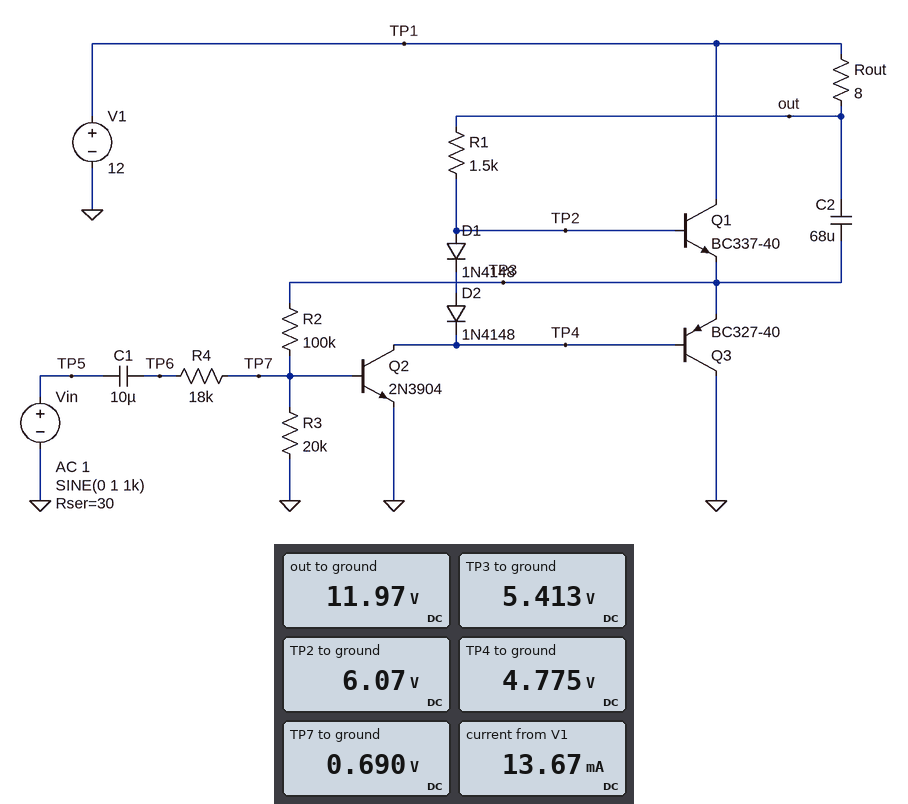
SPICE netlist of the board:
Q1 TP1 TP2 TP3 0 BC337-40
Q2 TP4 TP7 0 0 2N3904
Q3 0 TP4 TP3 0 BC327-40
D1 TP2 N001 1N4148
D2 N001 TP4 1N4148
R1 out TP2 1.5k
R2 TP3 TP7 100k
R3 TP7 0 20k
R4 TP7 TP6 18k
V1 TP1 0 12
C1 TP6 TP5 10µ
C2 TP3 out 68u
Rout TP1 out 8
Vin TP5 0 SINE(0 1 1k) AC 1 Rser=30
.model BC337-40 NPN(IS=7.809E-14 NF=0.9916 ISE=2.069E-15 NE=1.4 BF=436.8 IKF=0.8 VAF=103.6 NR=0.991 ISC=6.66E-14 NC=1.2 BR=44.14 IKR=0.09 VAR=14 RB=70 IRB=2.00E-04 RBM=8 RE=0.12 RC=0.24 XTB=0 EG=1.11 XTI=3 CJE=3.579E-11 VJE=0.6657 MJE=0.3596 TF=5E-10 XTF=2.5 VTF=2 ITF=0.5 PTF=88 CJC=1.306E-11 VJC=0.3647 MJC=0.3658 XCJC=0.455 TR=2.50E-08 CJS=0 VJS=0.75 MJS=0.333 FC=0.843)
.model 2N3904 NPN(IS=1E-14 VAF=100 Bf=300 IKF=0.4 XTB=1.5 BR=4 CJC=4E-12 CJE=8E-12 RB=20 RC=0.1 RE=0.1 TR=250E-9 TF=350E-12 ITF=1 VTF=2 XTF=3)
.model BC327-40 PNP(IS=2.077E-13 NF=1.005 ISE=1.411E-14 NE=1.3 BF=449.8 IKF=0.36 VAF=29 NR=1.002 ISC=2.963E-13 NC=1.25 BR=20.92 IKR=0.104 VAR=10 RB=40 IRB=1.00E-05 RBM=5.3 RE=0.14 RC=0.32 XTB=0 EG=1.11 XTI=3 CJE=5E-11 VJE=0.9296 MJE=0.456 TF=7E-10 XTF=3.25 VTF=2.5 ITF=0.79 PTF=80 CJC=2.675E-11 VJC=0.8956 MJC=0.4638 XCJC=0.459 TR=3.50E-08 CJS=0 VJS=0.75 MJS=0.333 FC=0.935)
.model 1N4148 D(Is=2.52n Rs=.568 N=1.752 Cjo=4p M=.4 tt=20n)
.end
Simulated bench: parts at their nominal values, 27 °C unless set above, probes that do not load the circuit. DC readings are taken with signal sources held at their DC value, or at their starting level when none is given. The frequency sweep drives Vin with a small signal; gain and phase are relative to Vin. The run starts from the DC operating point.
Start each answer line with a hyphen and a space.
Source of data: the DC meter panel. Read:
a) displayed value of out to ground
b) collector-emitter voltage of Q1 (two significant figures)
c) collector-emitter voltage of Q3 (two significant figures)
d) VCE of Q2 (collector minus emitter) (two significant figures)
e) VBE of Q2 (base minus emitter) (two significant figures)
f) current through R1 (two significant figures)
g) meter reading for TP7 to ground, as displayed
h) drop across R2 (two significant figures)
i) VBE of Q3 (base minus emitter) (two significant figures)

- 11.97 V
- 6.6 V
- -5.4 V
- 4.8 V
- 690 mV
- 3.9 mA
- 0.690 V
- 4.7 V
- -640 mV
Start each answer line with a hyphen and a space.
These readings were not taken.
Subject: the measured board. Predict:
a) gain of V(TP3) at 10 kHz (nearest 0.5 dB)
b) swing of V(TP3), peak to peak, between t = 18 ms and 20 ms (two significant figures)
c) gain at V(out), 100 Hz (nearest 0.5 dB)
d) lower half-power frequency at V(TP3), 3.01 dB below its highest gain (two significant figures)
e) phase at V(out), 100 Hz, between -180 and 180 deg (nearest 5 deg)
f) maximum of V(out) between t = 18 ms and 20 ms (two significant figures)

- 13.5 dB
- 8.6 V
- 3.0 dB
- 1.0 Hz
- -110 deg
- 16 V
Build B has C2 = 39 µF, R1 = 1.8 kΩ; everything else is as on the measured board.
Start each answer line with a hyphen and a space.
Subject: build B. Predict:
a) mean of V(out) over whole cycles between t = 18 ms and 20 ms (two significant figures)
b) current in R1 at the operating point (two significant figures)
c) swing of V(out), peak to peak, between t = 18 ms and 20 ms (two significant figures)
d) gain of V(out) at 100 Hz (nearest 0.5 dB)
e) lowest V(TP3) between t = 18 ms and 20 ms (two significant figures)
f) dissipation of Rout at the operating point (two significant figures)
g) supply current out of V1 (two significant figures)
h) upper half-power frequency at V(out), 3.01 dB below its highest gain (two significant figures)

- 12 V
- 3.4 mA
- 7.7 V
- -1.5 dB
- 1.0 V
- 92 µW
- 11 mA
- 590 kHz
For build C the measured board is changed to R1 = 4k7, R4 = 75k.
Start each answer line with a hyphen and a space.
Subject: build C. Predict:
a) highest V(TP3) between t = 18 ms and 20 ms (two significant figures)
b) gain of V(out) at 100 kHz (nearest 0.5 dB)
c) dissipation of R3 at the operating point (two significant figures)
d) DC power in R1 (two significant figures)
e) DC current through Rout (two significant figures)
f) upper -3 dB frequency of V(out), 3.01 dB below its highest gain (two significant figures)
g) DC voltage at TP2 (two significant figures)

- 5.6 V
- 0.5 dB
- 22 µW
- 10 mW
- 1.5 mA
- 350 kHz
- 5.1 V
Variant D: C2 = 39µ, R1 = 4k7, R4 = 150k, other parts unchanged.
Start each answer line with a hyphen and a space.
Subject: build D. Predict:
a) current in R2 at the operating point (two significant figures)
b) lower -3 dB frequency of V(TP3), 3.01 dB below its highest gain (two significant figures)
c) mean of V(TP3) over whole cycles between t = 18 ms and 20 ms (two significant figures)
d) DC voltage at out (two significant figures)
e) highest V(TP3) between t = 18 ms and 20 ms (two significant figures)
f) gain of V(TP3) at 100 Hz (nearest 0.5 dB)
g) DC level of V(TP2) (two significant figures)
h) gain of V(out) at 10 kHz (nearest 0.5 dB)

- 38 µA
- 110 mHz
- 4.5 V
- 12 V
- 5.0 V
- -4.5 dB
- 5.1 V
- -5.5 dB
